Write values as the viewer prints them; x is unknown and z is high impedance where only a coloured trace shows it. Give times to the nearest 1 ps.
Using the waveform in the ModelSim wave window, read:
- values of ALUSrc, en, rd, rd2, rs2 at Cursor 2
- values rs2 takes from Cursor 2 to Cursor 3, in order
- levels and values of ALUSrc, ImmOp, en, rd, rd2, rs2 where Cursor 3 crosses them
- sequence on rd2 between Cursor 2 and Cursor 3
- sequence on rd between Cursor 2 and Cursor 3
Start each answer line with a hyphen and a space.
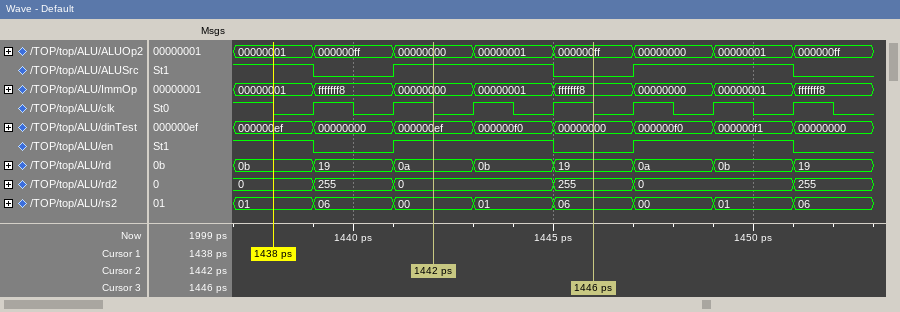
- ALUSrc=1, en=1, rd=0a, rd2=0, rs2=00
- 00, 01, 06
- ALUSrc=0, ImmOp=fffffff8, en=0, rd=19, rd2=255, rs2=06
- 0, 255
- 0a, 0b, 19
